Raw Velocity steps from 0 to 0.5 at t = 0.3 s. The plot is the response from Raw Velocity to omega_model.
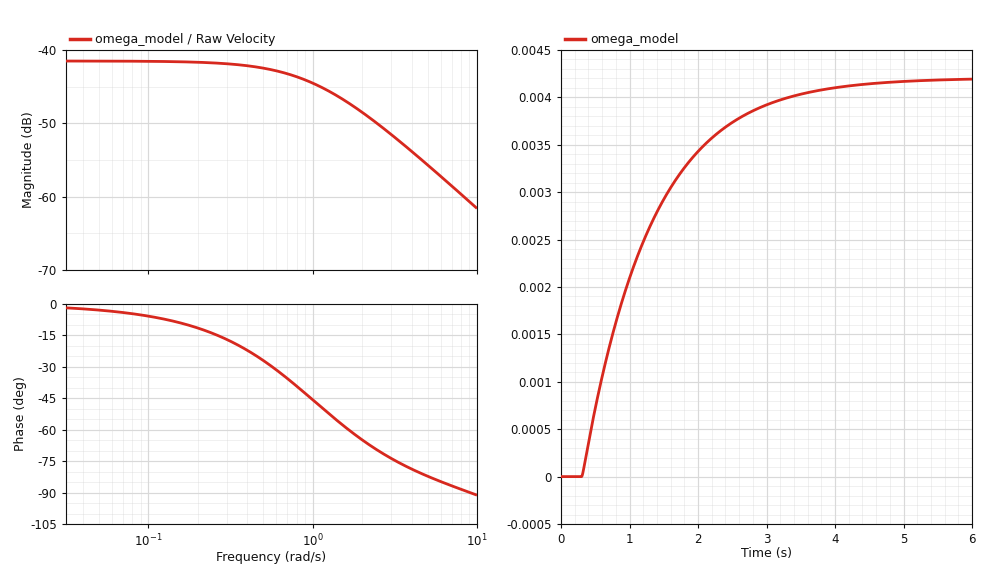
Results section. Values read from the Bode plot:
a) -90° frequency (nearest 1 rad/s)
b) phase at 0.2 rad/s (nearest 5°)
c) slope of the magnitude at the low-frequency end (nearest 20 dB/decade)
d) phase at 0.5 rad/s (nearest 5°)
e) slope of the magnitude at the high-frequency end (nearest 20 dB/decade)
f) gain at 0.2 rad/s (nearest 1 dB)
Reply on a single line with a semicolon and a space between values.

9 rad/s; -10°; 0 dB/decade; -25°; -20 dB/decade; -42 dB
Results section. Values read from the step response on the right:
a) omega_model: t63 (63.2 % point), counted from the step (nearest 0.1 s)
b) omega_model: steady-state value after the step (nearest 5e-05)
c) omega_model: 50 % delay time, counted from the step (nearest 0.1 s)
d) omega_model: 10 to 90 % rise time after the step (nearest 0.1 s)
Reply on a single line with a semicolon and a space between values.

1.0 s; 0.00420; 0.7 s; 2.2 s
